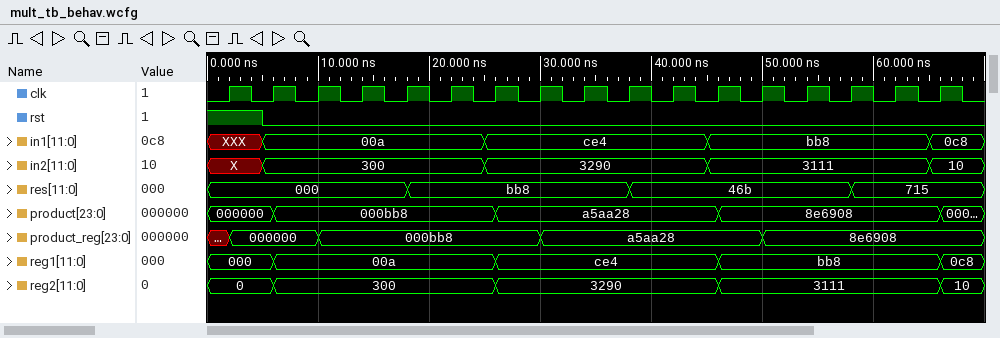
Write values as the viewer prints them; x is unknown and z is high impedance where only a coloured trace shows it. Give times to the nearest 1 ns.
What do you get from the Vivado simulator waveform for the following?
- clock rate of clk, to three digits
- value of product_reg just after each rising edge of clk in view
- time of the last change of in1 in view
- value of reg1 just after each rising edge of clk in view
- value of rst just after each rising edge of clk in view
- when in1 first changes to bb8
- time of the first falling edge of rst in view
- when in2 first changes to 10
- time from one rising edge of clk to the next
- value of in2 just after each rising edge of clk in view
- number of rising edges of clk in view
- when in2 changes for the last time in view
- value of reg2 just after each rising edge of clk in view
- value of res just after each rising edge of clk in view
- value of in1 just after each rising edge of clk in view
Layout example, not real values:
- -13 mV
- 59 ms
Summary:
- 250 MHz
- 000000, 000000, 000bb8, 000bb8, 000bb8, 000bb8, 000bb8, a5aa28, a5aa28, a5aa28, a5aa28, a5aa28, 8e6908, 8e6908, 8e6908, 8e6908, 8e6908
- 65 ns
- 000, 00a, 00a, 00a, 00a, 00a, ce4, ce4, ce4, ce4, ce4, bb8, bb8, bb8, bb8, bb8, 0c8
- 1 0 0 0 0 0 0 0 0 0 0 0 0 0 0 0 0
- 45 ns
- 5 ns
- 65 ns
- 4 ns
- X, 300, 300, 300, 300, 300, 3290, 3290, 3290, 3290, 3290, 3111, 3111, 3111, 3111, 3111, 10
- 17
- 65 ns
- 0, 300, 300, 300, 300, 300, 3290, 3290, 3290, 3290, 3290, 3111, 3111, 3111, 3111, 3111, 10
- 000, 000, 000, 000, bb8, bb8, bb8, bb8, bb8, 46b, 46b, 46b, 46b, 46b, 715, 715, 715
- XXX, 00a, 00a, 00a, 00a, 00a, ce4, ce4, ce4, ce4, ce4, bb8, bb8, bb8, bb8, bb8, 0c8
